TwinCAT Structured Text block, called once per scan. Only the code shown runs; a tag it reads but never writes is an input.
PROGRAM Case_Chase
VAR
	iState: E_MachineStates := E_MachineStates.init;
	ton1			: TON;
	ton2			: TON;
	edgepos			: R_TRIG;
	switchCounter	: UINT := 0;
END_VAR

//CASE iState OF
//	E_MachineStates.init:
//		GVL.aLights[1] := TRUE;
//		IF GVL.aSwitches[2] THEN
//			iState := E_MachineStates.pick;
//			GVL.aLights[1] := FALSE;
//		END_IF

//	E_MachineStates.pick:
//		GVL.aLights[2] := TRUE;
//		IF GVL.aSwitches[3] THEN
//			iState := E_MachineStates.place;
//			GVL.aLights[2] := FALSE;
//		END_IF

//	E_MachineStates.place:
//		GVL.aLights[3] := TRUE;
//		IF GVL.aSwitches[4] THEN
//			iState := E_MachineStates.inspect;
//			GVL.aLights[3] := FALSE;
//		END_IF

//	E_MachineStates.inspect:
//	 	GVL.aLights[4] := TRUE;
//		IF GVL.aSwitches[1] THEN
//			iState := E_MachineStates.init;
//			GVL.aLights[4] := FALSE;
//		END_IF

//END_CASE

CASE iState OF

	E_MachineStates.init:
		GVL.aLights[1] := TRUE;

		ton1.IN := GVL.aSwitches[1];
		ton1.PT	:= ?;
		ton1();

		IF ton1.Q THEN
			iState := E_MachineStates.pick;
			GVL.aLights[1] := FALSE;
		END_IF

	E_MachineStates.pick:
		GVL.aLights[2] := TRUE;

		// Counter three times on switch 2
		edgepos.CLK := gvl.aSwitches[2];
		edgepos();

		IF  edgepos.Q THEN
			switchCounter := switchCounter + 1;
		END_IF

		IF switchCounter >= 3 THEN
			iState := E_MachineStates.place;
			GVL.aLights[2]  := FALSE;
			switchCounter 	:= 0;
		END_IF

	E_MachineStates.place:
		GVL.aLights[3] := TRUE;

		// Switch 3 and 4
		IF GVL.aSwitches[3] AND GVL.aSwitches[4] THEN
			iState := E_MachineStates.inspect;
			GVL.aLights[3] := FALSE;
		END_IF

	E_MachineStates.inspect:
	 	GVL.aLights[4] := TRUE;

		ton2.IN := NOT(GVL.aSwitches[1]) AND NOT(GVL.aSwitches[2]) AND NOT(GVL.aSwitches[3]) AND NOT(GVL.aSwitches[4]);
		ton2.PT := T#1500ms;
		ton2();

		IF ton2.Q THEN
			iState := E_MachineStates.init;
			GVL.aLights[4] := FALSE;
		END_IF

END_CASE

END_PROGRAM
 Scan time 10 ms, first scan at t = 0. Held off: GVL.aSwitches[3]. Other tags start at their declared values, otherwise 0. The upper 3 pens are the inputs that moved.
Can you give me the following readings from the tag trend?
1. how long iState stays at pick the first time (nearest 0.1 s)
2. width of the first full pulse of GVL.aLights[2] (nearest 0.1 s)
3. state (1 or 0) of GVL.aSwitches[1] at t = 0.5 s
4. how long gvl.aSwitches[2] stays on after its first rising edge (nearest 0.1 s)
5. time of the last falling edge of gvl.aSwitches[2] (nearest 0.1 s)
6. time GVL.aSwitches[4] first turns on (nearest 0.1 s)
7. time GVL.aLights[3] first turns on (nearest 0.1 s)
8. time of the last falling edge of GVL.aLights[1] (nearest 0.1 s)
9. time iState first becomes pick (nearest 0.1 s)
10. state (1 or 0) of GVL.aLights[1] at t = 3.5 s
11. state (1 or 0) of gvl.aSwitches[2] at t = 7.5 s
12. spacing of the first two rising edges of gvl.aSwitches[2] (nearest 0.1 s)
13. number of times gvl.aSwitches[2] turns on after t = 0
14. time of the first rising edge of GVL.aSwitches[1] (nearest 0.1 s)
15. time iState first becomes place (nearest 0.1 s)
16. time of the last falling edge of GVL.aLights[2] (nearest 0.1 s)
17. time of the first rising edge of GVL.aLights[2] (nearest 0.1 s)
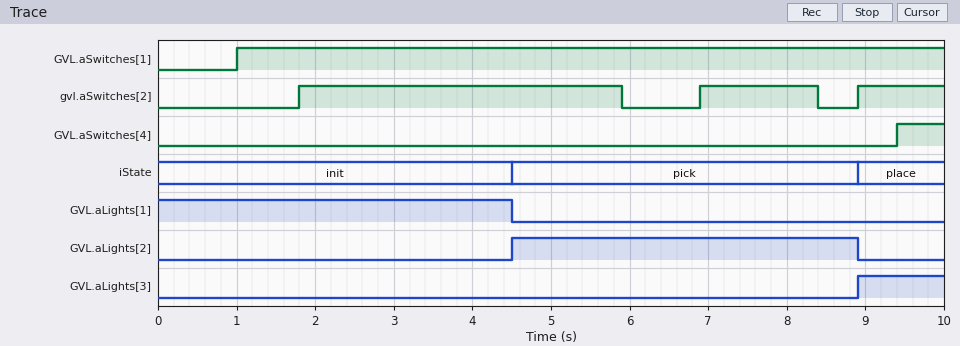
4.4 s
4.4 s
0
4.1 s
8.4 s
9.4 s
8.9 s
4.5 s
4.5 s
1
1
5.1 s
3
1.0 s
8.9 s
8.9 s
4.5 s
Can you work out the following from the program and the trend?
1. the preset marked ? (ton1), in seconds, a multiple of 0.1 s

3.5 s
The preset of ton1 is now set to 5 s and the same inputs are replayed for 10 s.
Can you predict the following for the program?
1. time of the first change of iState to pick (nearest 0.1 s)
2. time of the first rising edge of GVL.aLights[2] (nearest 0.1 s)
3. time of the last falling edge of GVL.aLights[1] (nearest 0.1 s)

6.0 s
6.0 s
6.0 s
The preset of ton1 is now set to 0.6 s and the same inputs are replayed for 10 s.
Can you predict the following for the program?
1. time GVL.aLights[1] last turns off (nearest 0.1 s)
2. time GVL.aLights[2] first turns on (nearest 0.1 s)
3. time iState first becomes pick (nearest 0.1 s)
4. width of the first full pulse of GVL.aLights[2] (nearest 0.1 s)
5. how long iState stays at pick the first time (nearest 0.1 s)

1.6 s
1.6 s
1.6 s
7.3 s
7.3 s
